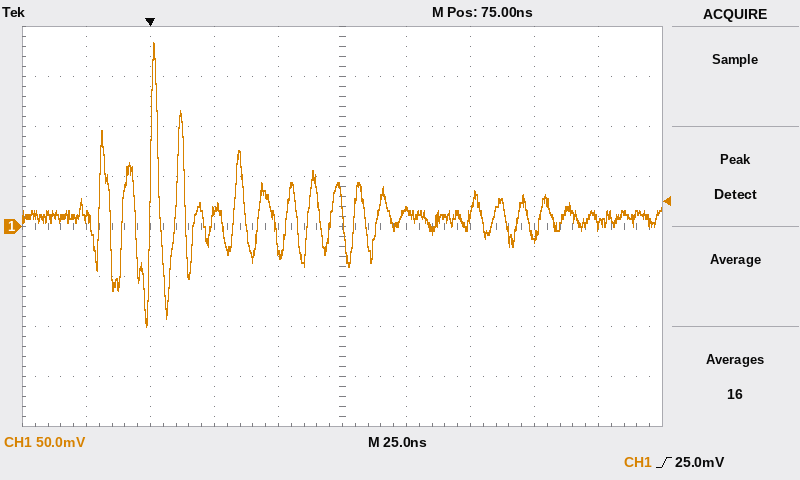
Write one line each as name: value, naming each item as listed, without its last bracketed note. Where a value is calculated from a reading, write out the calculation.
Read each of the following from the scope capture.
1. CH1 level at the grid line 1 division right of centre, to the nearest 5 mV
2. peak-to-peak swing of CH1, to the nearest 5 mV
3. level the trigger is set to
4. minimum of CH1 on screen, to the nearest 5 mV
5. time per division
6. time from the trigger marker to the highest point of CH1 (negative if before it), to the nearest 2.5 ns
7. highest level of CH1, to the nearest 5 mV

CH1 level at the grid line 1 division right of centre, to the nearest 5 mV: 15 mV
peak-to-peak swing of CH1, to the nearest 5 mV: 185 mV − (-100 mV) = 285 mV
level the trigger is set to: 25.0 mV
minimum of CH1 on screen, to the nearest 5 mV: -100 mV
time per division: 25 ns
time from the trigger marker to the highest point of CH1 (negative if before it), to the nearest 2.5 ns: +2.5 ns
highest level of CH1, to the nearest 5 mV: 185 mV
